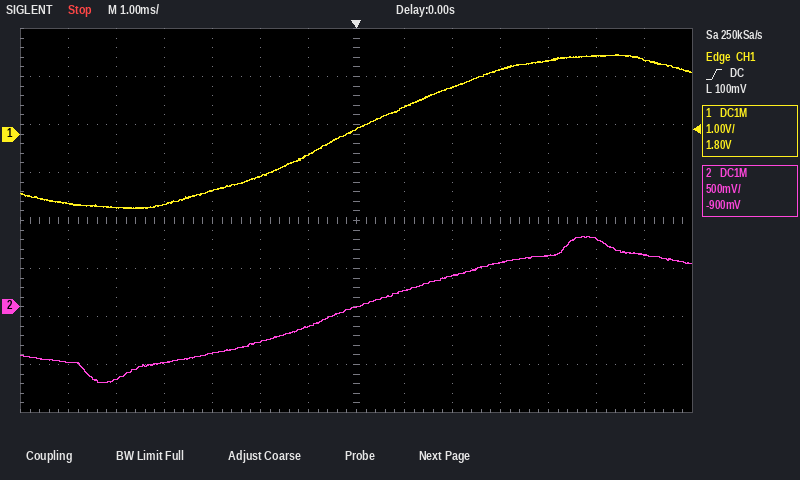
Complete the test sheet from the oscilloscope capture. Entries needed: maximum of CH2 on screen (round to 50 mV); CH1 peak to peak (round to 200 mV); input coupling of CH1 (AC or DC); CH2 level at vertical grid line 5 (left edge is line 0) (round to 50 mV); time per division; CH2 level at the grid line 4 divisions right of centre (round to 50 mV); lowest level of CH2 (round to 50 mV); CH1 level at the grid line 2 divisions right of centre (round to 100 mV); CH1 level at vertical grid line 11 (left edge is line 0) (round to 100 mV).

750 mV
3.2 V
DC
-350 mV
1 ms
550 mV
-800 mV
1.0 V
1.5 V
